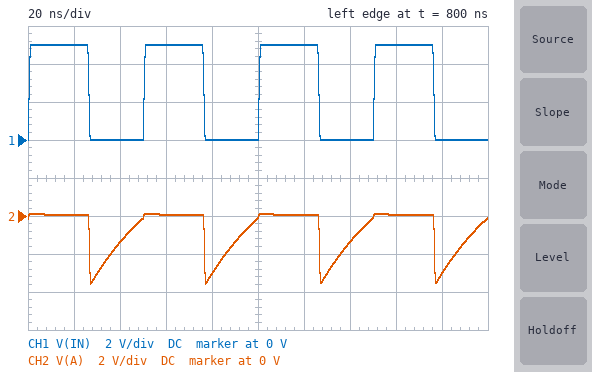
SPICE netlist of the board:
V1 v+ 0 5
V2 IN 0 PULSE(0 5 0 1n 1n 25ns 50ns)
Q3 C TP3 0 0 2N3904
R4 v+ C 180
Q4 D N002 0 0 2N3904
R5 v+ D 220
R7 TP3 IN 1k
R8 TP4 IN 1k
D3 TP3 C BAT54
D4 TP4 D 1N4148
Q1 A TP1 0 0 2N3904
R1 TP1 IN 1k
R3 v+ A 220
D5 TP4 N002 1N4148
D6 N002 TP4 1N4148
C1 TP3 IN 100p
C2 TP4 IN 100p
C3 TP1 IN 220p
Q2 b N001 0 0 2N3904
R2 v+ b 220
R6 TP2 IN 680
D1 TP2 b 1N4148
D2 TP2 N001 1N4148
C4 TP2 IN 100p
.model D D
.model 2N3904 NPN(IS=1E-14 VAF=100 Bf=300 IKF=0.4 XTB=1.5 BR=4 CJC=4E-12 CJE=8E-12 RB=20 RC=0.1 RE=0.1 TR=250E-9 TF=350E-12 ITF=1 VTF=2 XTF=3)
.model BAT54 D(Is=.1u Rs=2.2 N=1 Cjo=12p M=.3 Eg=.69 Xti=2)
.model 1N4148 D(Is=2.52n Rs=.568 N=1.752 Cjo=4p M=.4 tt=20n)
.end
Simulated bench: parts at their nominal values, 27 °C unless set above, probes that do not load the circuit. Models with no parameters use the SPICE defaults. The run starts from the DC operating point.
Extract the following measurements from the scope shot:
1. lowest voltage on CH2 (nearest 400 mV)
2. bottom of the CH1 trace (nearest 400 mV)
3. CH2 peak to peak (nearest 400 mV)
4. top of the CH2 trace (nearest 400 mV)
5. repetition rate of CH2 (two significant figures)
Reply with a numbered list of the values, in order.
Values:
1. -3.6 V
2. 0 V
3. 3.6 V
4. 0 V
5. 20 MHz
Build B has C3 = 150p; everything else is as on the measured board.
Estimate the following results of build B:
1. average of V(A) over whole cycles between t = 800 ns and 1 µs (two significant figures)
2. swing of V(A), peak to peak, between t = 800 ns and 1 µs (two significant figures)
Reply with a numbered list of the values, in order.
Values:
1. -500 mV
2. 3.6 V
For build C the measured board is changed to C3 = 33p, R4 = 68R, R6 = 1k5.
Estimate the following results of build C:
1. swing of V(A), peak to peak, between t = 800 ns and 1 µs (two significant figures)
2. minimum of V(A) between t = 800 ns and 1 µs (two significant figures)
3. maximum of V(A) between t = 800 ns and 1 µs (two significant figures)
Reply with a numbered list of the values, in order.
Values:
1. 2.4 V
2. -2.3 V
3. 110 mV
